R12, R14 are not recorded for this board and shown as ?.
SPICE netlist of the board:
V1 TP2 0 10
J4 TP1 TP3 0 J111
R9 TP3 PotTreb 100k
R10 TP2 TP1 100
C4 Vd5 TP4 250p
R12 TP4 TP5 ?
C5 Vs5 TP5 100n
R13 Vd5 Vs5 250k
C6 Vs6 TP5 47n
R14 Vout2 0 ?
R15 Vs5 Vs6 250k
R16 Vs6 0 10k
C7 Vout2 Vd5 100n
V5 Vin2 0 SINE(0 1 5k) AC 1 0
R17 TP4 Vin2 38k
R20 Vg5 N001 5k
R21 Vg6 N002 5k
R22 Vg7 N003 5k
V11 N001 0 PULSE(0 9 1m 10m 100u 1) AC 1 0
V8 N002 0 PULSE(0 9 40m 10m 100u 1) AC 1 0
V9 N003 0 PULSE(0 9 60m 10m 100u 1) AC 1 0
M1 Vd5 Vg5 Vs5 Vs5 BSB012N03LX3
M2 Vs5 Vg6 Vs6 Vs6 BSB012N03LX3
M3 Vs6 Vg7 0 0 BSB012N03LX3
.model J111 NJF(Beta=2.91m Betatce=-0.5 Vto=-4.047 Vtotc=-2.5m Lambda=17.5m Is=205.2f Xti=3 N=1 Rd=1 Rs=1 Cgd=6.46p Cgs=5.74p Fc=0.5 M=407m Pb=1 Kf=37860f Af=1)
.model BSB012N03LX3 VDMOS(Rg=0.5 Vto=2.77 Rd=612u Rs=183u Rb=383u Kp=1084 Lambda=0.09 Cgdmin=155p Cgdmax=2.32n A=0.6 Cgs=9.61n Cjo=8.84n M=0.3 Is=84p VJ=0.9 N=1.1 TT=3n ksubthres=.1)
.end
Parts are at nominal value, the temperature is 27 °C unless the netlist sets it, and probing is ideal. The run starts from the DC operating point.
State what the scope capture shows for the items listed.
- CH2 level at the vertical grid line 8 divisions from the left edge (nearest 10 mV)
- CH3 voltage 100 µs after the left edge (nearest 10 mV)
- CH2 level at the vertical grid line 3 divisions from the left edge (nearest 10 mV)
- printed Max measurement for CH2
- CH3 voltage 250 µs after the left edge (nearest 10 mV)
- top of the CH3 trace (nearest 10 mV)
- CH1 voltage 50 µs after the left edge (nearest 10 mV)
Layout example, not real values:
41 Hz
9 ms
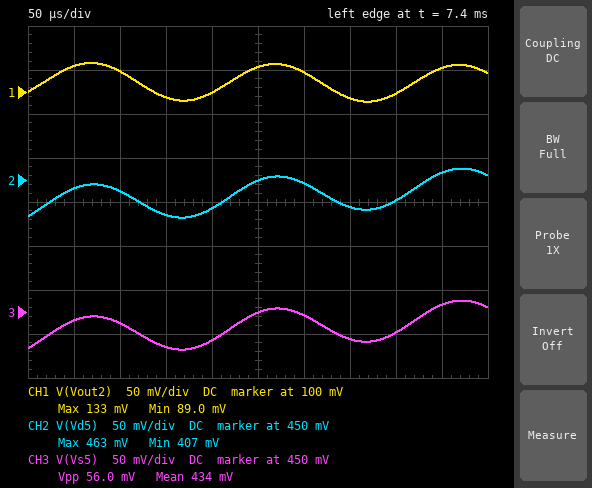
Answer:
430 mV
440 mV
410 mV
463 mV
450 mV
460 mV
130 mV
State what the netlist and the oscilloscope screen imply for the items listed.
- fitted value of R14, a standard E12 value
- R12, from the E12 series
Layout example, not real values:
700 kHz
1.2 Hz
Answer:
22 kΩ
47 kΩ
